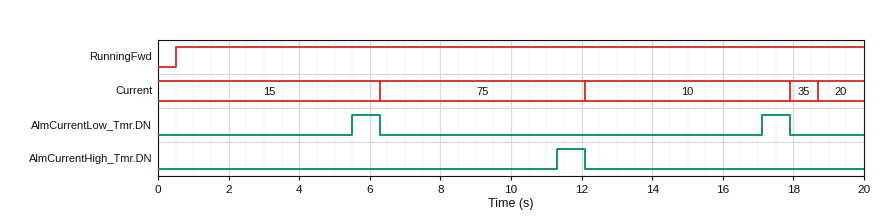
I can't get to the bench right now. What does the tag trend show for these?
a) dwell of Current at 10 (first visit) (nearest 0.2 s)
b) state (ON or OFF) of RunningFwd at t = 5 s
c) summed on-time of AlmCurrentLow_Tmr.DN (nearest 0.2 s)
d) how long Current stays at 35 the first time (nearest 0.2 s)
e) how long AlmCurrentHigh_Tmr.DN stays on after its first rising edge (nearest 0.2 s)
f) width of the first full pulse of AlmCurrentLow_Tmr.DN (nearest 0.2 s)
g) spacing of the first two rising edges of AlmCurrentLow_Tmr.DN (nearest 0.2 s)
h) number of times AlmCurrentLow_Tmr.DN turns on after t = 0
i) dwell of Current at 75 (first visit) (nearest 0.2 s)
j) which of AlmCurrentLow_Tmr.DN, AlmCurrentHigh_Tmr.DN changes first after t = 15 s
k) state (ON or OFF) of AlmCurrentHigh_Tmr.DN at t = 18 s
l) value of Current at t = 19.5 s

5.8 s
ON
1.6 s
0.8 s
0.8 s
0.8 s
11.6 s
2
5.8 s
AlmCurrentLow_Tmr.DN
OFF
20
